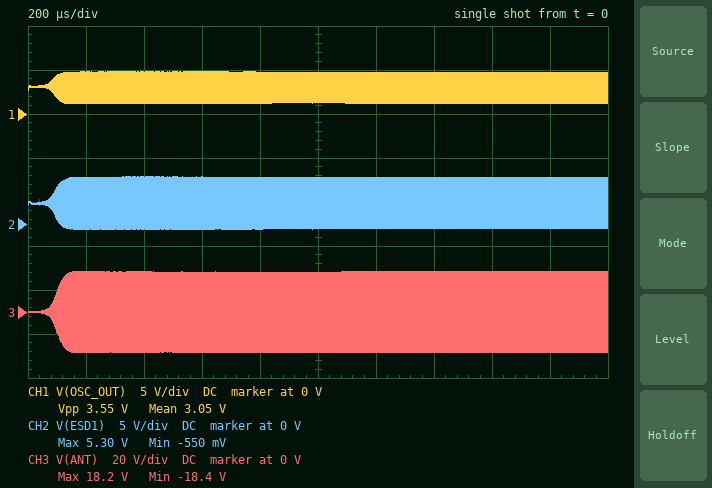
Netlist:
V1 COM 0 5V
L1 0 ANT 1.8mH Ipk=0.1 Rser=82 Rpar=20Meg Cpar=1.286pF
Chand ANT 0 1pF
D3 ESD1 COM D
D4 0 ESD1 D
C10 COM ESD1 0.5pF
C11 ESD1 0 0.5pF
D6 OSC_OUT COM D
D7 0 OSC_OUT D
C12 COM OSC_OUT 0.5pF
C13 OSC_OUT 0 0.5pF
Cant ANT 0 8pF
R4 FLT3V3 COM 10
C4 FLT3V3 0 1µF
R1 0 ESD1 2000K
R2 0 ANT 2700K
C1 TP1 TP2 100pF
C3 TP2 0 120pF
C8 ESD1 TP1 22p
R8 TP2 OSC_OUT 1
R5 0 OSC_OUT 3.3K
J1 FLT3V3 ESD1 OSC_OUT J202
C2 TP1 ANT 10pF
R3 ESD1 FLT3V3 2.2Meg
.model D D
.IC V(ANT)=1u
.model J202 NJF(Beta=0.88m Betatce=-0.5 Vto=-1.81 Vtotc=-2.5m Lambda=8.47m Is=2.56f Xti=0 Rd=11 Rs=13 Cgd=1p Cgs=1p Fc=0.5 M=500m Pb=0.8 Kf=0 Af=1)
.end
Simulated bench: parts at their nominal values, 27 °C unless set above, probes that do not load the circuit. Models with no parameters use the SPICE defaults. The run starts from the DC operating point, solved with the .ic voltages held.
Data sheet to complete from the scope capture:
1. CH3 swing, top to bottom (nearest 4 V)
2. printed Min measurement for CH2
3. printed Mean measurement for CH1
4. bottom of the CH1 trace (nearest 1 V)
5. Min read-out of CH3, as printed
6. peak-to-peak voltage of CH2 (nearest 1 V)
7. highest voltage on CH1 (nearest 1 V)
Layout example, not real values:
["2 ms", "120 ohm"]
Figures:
["36 V", "-550 mV", "3.05 V", "1 V", "-18.4 V", "6 V", "5 V"]
